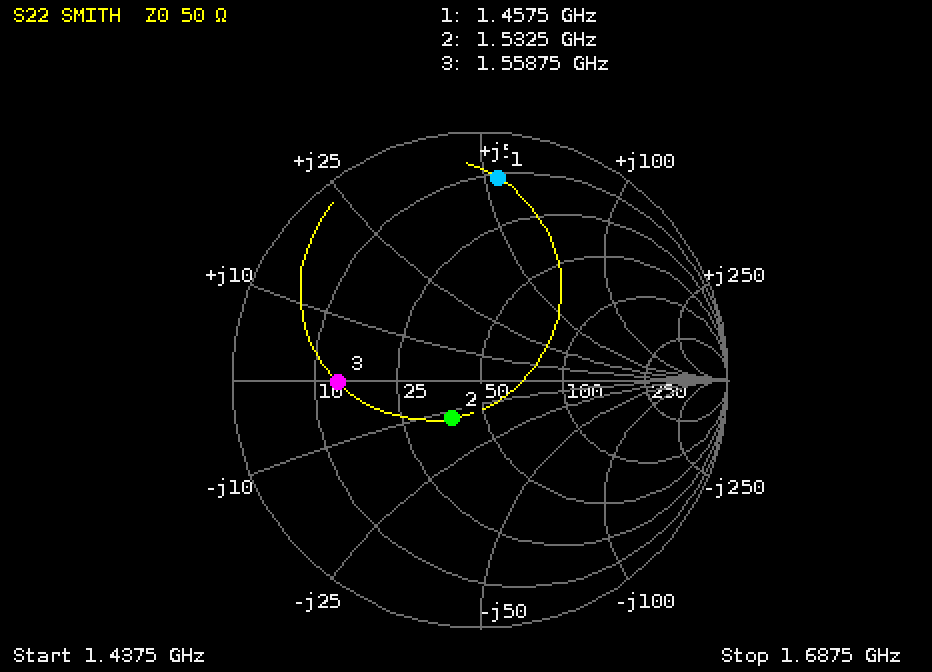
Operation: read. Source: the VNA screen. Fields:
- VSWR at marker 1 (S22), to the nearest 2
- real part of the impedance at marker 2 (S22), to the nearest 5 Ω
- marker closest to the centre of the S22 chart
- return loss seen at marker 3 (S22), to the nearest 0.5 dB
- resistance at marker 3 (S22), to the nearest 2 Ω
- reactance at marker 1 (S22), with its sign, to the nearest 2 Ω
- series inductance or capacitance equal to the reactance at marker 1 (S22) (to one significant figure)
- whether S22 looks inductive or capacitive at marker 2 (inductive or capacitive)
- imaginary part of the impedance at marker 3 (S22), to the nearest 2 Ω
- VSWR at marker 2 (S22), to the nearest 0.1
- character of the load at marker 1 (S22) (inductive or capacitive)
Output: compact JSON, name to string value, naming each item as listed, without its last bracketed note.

{"VSWR at marker 1 (S22), to the nearest 2": "10", "real part of the impedance at marker 2 (S22), to the nearest 5 Ω": "40 Ω", "marker closest to the centre of the S22 chart": "marker 2", "return loss seen at marker 3 (S22), to the nearest 0.5 dB": "5.0 dB", "resistance at marker 3 (S22), to the nearest 2 Ω": "14 Ω", "reactance at marker 1 (S22), with its sign, to the nearest 2 Ω": "+54 Ω", "series inductance or capacitance equal to the reactance at marker 1 (S22)": "6 nH", "whether S22 looks inductive or capacitive at marker 2": "capacitive", "imaginary part of the impedance at marker 3 (S22), to the nearest 2 Ω": "0 Ω", "VSWR at marker 2 (S22), to the nearest 0.1": "1.5", "character of the load at marker 1 (S22)": "inductive"}
